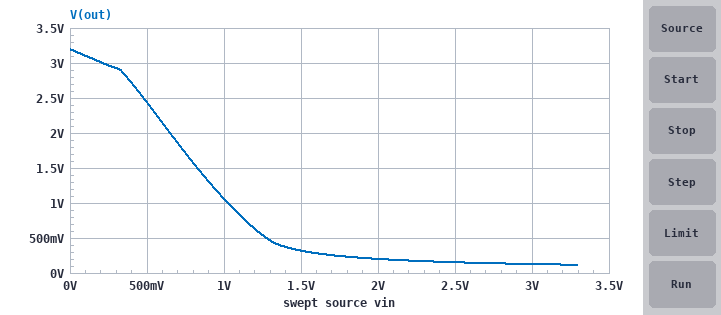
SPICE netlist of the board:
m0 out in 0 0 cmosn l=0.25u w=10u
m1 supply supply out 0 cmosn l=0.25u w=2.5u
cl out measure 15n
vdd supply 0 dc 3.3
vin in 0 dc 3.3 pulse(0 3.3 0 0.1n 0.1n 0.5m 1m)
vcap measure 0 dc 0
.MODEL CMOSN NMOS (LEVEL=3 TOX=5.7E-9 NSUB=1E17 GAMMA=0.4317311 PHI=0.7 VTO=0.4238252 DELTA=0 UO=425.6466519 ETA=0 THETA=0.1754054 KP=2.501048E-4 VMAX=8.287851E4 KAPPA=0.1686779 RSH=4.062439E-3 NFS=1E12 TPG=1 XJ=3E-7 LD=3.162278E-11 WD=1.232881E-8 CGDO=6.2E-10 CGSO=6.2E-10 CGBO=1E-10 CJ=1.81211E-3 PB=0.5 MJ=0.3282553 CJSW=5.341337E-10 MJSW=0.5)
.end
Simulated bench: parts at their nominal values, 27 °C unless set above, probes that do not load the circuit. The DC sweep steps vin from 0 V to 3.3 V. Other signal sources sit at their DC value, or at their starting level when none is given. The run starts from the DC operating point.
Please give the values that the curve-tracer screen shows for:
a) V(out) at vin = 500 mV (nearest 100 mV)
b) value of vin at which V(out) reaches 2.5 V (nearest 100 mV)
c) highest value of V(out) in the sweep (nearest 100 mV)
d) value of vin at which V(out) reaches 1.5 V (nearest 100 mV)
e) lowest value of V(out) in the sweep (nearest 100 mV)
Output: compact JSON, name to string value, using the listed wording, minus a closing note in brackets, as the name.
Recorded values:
{"V(out) at vin = 500 mV": "2.4 V", "value of vin at which V(out) reaches 2.5 V": "500 mV", "highest value of V(out) in the sweep": "3.2 V", "value of vin at which V(out) reaches 1.5 V": "800 mV", "lowest value of V(out) in the sweep": "100 mV"}
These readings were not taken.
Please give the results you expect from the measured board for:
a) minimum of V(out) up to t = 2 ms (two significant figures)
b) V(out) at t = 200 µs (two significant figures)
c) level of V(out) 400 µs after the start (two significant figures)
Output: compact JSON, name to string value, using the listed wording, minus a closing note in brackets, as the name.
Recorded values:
{"minimum of V(out) up to t = 2 ms": "120 mV", "V(out) at t = 200 µs": "120 mV", "level of V(out) 400 µs after the start": "120 mV"}
